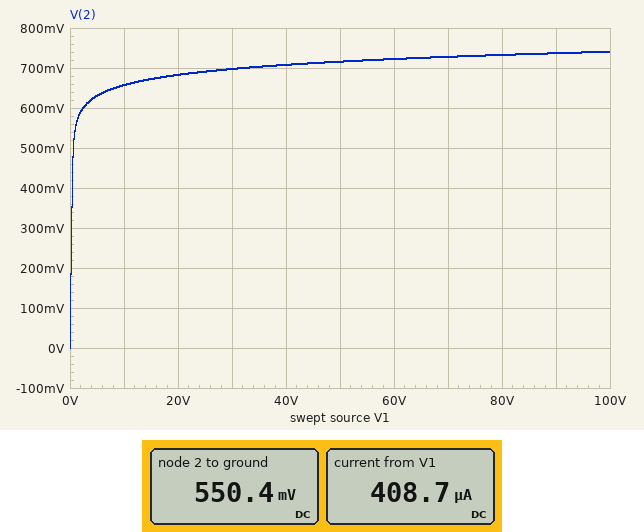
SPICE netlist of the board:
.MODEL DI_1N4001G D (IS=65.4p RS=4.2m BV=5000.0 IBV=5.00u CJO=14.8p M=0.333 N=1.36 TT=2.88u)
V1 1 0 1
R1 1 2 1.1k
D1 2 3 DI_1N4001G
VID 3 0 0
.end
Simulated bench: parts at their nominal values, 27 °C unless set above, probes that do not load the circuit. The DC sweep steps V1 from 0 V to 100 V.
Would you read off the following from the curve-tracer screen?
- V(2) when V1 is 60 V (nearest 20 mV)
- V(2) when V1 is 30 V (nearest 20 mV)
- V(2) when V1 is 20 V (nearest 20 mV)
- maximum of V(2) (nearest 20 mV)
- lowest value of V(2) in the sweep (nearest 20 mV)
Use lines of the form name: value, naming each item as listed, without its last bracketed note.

V(2) when V1 is 60 V: 720 mV
V(2) when V1 is 30 V: 700 mV
V(2) when V1 is 20 V: 680 mV
maximum of V(2): 740 mV
lowest value of V(2) in the sweep: 0 V
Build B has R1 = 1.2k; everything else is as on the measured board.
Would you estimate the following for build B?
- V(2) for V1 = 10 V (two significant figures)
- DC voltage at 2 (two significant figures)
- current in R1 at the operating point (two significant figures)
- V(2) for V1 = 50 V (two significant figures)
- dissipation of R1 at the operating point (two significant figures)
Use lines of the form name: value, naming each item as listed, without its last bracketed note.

V(2) for V1 = 10 V: 650 mV
DC voltage at 2: 550 mV
current in R1 at the operating point: 380 µA
V(2) for V1 = 50 V: 710 mV
dissipation of R1 at the operating point: 170 µW
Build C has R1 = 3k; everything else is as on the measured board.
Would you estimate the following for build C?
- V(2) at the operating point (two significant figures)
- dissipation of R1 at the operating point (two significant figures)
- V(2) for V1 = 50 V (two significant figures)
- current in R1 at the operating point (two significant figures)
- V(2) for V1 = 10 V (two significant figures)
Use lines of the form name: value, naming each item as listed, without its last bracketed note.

V(2) at the operating point: 520 mV
dissipation of R1 at the operating point: 78 µW
V(2) for V1 = 50 V: 680 mV
current in R1 at the operating point: 160 µA
V(2) for V1 = 10 V: 620 mV
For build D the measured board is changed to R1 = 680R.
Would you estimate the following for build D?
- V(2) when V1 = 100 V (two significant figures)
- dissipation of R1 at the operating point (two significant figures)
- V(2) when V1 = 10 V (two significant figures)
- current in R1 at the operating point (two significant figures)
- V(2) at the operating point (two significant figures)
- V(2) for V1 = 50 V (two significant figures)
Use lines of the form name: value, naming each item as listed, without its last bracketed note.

V(2) when V1 = 100 V: 760 mV
dissipation of R1 at the operating point: 280 µW
V(2) when V1 = 10 V: 670 mV
current in R1 at the operating point: 640 µA
V(2) at the operating point: 570 mV
V(2) for V1 = 50 V: 730 mV
